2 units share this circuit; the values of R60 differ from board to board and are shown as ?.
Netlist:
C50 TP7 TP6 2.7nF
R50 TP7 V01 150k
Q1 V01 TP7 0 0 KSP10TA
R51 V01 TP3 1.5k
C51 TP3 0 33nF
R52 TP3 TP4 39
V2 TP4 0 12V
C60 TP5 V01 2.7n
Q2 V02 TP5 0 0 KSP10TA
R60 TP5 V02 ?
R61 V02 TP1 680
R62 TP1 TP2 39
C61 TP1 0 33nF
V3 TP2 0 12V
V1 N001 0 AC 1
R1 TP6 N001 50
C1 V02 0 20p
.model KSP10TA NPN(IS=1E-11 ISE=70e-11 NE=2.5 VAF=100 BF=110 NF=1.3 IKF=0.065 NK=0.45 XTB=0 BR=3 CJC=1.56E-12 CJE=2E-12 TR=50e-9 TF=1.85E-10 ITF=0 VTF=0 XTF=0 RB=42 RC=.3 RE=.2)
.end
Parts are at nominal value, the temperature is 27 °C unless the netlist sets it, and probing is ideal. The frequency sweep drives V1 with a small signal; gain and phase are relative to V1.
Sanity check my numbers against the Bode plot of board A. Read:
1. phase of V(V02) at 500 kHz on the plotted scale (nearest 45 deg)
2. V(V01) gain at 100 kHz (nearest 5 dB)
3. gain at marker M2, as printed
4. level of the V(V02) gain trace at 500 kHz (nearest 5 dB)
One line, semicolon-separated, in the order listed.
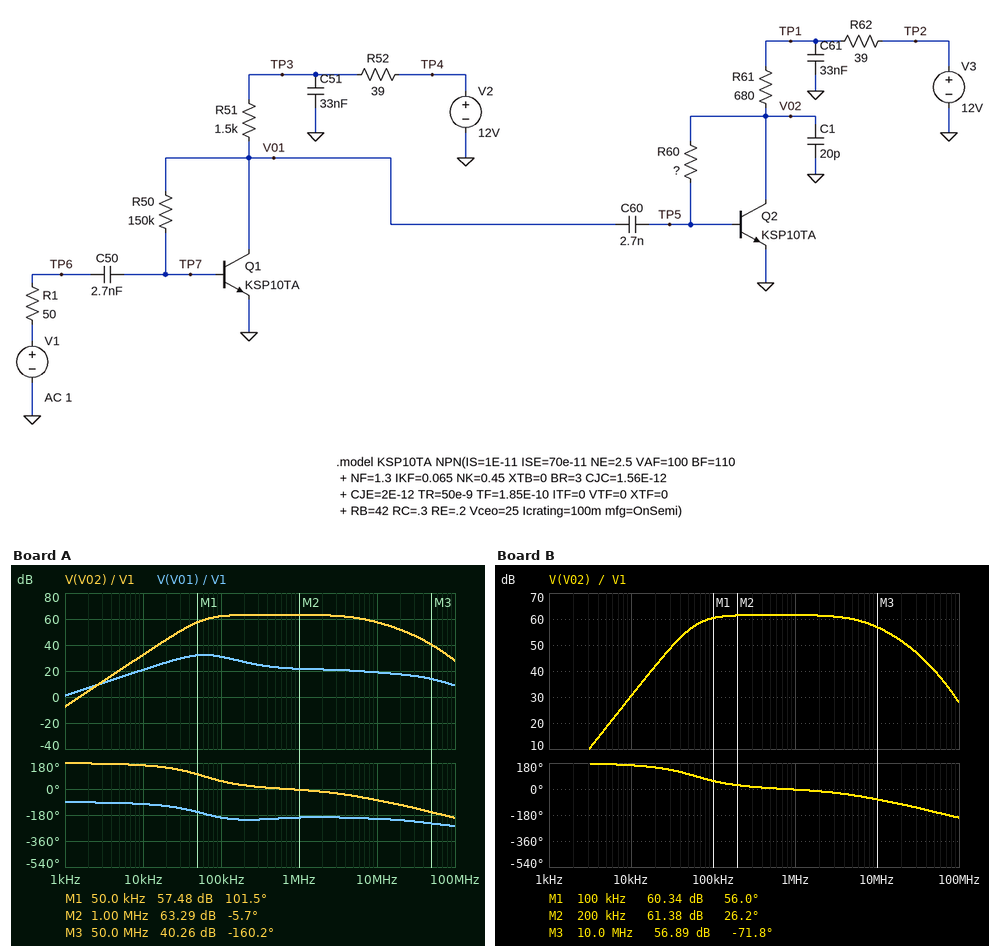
0 deg; 30 dB; 63.29 dB; 65 dB
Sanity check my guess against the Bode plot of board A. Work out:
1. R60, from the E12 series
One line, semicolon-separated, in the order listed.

39 kΩ
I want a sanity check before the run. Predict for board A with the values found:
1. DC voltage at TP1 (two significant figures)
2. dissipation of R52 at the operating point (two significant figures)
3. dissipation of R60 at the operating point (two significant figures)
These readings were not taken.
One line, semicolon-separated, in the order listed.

12 V; 360 µW; 570 µW
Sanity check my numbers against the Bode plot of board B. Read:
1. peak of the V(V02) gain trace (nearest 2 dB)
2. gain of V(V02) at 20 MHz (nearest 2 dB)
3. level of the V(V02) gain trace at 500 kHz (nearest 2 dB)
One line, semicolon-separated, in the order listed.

62 dB; 52 dB; 62 dB
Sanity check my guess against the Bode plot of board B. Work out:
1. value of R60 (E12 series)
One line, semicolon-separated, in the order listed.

27 kΩ
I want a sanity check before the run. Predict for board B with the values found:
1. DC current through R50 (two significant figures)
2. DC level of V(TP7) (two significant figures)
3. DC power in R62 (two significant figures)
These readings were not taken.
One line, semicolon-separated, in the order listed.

44 µA; 660 mV; 4.3 mW
